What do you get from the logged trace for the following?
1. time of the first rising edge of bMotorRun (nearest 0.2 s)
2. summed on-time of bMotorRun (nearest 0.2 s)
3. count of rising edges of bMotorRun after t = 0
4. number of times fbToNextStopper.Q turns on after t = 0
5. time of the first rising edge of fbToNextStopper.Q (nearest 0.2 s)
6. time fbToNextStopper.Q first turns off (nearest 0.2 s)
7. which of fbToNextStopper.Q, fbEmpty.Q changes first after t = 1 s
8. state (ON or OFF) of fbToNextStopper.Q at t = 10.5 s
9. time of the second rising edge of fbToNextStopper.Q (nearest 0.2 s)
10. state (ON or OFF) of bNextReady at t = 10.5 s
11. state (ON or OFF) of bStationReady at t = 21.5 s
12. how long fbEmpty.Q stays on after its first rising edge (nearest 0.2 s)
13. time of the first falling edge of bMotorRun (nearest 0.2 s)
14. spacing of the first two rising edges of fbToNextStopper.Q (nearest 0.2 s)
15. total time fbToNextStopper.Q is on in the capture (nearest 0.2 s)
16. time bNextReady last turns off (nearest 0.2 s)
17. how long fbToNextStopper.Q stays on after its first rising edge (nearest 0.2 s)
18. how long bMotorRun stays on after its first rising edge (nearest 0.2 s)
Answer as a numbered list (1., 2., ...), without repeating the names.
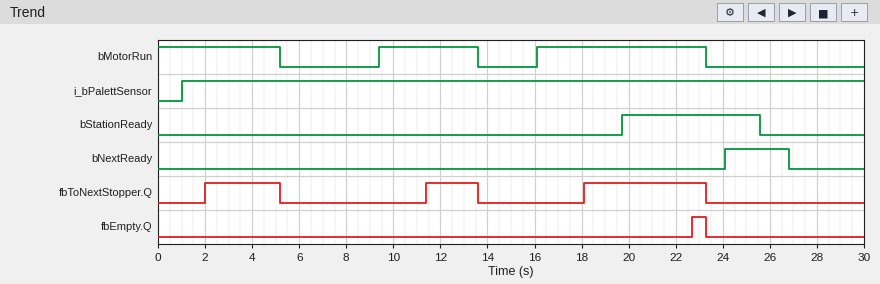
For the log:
1. 9.4 s
2. 16.6 s
3. 2
4. 3
5. 2.0 s
6. 5.2 s
7. fbToNextStopper.Q
8. OFF
9. 11.4 s
10. OFF
11. ON
12. 0.6 s
13. 5.2 s
14. 9.4 s
15. 10.6 s
16. 26.8 s
17. 3.2 s
18. 4.2 s
